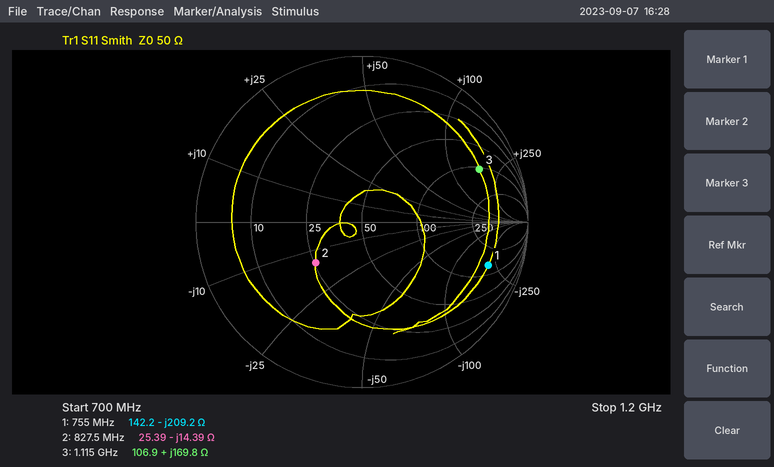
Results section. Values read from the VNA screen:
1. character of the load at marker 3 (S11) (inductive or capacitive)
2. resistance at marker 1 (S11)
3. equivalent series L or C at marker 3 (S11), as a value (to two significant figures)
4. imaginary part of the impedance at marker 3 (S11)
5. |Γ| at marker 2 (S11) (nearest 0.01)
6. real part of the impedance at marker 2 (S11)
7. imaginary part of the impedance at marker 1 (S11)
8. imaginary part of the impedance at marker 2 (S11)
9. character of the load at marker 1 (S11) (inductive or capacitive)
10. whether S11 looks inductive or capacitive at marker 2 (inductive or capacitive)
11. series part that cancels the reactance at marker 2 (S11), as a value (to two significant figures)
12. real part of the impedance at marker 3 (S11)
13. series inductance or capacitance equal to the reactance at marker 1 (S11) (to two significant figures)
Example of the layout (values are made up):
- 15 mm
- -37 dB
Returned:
- inductive
- 142.2 Ω
- 24 nH
- +169.8 Ω
- 0.37
- 25.39 Ω
- -209.2 Ω
- -14.39 Ω
- capacitive
- capacitive
- 2.8 nH
- 106.9 Ω
- 1.0 pF
